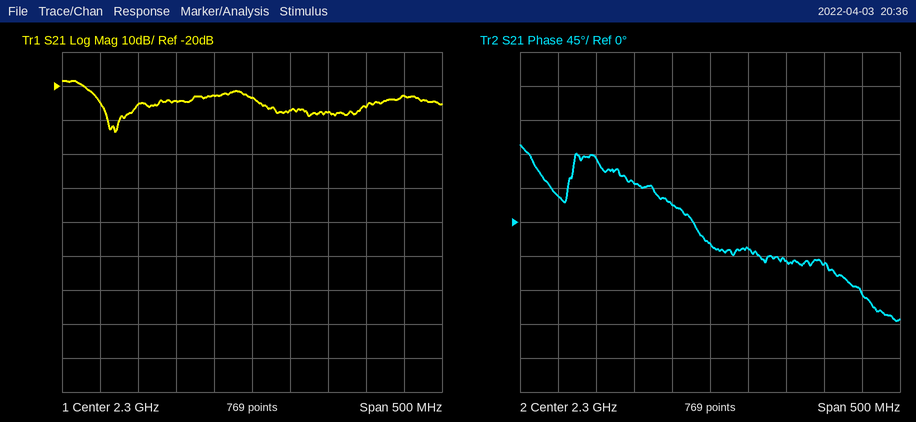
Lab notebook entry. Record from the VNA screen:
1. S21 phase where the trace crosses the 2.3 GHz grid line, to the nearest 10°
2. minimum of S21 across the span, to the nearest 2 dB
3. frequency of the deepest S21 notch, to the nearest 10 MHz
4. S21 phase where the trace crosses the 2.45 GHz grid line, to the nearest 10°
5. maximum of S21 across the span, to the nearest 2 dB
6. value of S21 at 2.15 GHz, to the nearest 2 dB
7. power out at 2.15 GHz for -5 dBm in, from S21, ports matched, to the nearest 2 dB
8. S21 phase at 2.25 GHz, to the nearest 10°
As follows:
-30°
-34 dB
2.12 GHz
-60°
-18 dB
-26 dB
-30 dBm
20°
